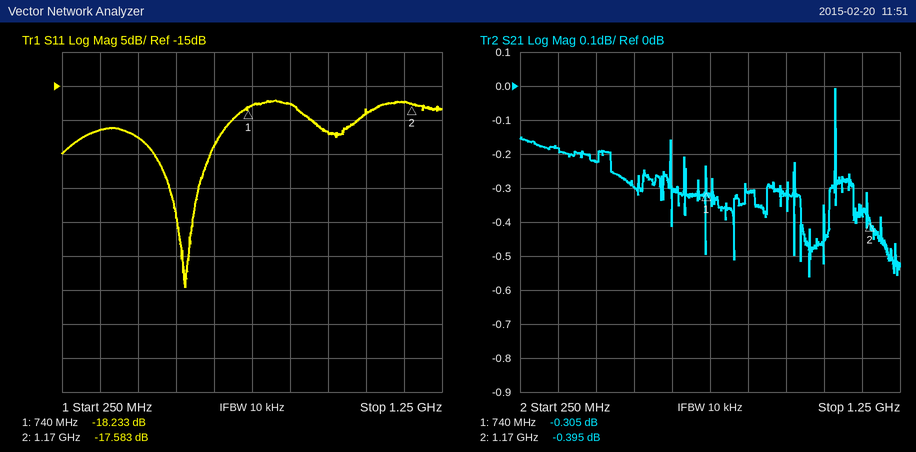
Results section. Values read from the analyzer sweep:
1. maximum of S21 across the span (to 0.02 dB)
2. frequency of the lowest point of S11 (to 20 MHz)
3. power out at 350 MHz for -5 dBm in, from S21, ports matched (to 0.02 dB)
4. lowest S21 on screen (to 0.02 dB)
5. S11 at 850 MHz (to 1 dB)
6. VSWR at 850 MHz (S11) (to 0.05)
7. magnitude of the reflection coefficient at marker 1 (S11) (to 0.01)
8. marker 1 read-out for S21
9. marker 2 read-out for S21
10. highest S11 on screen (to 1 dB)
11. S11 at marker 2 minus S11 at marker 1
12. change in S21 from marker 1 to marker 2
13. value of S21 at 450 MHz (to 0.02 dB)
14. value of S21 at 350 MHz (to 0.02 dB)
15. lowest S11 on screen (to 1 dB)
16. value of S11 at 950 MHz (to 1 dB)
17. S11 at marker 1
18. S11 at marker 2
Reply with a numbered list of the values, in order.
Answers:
1. 0.00 dB
2. 580 MHz
3. -5.18 dBm
4. -0.56 dB
5. -18 dB
6. 1.30
7. 0.12
8. -0.305 dB
9. -0.395 dB
10. -17 dB
11. 0.650 dB
12. -0.090 dB
13. -0.22 dB
14. -0.18 dB
15. -45 dB
16. -22 dB
17. -18.233 dB
18. -17.583 dB
